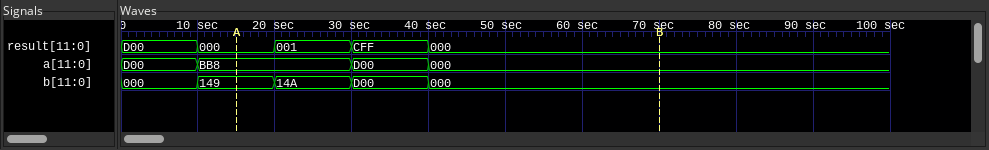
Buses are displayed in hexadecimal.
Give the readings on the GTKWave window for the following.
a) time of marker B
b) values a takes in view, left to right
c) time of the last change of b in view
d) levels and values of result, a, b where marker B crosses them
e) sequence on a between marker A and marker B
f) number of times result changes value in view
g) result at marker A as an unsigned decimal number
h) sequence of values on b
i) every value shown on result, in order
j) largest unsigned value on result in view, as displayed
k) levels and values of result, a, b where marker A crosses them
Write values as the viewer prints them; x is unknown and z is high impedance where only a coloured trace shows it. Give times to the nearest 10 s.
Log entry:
70 s
D00, BB8, D00, 000
40 s
result=000, a=000, b=000
BB8, D00, 000
4
0
000, 149, 14A, D00, 000
D00, 000, 001, CFF, 000
D00
result=000, a=BB8, b=149
